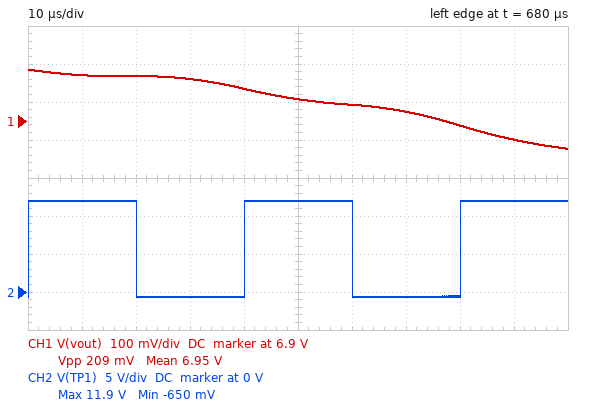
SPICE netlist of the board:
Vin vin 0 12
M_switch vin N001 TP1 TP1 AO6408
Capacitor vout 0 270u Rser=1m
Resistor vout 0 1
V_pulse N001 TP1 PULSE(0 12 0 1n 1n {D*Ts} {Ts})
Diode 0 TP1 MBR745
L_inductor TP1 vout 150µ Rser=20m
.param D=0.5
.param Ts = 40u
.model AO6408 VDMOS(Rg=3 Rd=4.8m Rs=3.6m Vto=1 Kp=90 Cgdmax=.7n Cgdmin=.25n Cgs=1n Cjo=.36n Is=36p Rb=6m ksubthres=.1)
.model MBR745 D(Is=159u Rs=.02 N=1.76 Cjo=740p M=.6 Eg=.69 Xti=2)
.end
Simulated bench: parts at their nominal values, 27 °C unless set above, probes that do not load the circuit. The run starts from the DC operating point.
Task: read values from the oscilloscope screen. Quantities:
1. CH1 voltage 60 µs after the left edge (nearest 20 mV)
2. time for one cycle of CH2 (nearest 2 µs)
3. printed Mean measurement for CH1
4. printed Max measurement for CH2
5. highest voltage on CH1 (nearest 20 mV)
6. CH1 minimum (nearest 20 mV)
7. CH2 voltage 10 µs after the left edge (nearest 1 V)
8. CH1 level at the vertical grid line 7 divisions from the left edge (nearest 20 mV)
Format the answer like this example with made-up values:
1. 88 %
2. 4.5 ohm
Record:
1. 6.94 V
2. 40 µs
3. 6.95 V
4. 11.9 V
5. 7.04 V
6. 6.82 V
7. 12 V
8. 6.92 V
